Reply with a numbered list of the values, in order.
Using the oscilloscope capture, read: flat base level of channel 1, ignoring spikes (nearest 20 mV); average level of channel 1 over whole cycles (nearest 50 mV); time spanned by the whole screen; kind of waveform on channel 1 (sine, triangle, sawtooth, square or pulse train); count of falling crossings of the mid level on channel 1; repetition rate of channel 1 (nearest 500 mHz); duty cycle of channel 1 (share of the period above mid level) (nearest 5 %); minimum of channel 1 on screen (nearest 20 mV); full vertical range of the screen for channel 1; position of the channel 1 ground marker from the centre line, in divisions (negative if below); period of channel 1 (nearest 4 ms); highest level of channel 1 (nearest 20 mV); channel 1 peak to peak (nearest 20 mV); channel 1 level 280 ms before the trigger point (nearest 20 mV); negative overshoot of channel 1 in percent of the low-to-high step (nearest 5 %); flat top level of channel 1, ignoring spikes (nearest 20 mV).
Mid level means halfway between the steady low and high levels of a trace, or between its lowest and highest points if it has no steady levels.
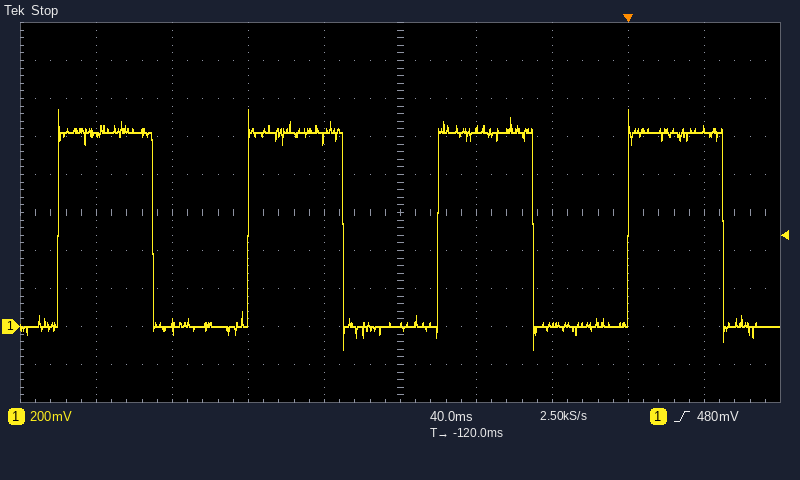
1. 0 mV
2. 500 mV
3. 400 ms
4. square
5. 4
6. 10.0 Hz
7. 50 %
8. -120 mV
9. 2 V
10. -3.0 div
11. 100 ms
12. 1.14 V
13. 1.26 V
14. 1.02 V
15. 10 %
16. 1.02 V
